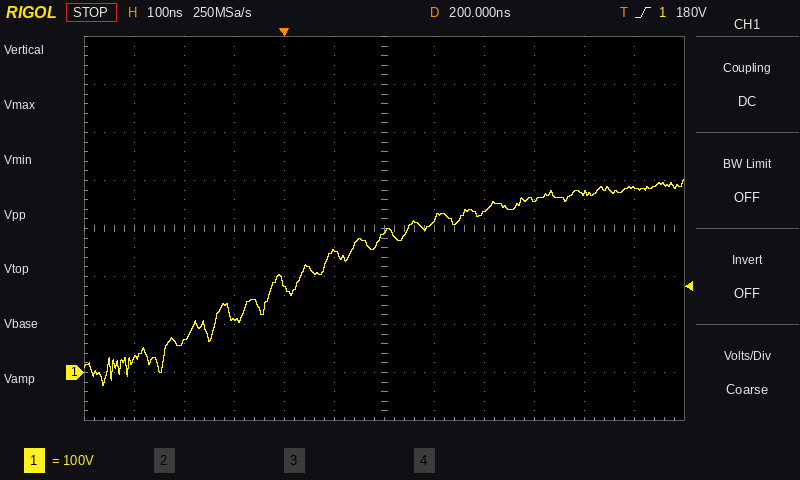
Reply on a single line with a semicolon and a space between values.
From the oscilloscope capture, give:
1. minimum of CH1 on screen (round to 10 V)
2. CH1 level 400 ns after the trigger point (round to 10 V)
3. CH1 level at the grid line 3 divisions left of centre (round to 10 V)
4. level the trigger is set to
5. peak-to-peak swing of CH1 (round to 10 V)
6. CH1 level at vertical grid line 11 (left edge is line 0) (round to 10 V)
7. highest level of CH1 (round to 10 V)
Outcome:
-30 V; 330 V; 110 V; 180 V; 430 V; 390 V; 400 V
